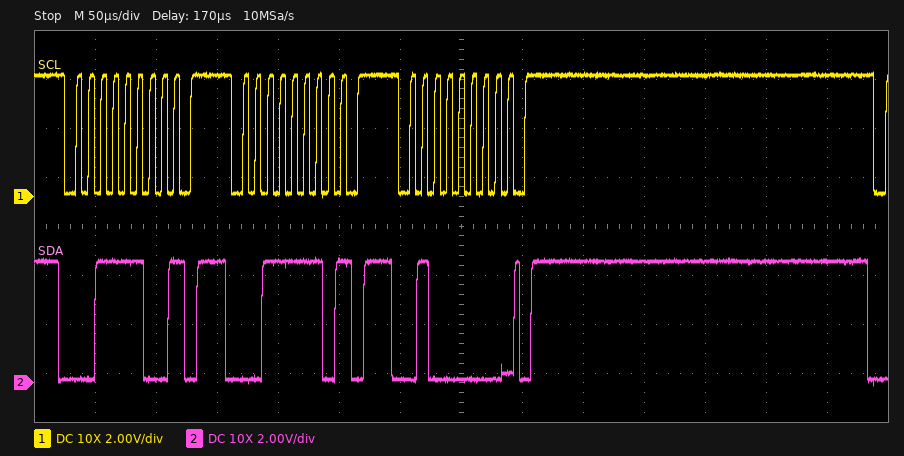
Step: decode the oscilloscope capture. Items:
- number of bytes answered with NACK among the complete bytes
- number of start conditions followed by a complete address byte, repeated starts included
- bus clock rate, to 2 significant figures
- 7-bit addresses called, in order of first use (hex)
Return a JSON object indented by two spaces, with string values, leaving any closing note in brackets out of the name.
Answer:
{
  "number of bytes answered with NACK among the complete bytes": "2",
  "number of start conditions followed by a complete address byte, repeated starts included": "3",
  "bus clock rate, to 2 significant figures": "100 kHz",
  "7-bit addresses called, in order of first use": "0x1E 0x1F 0x20"
}
